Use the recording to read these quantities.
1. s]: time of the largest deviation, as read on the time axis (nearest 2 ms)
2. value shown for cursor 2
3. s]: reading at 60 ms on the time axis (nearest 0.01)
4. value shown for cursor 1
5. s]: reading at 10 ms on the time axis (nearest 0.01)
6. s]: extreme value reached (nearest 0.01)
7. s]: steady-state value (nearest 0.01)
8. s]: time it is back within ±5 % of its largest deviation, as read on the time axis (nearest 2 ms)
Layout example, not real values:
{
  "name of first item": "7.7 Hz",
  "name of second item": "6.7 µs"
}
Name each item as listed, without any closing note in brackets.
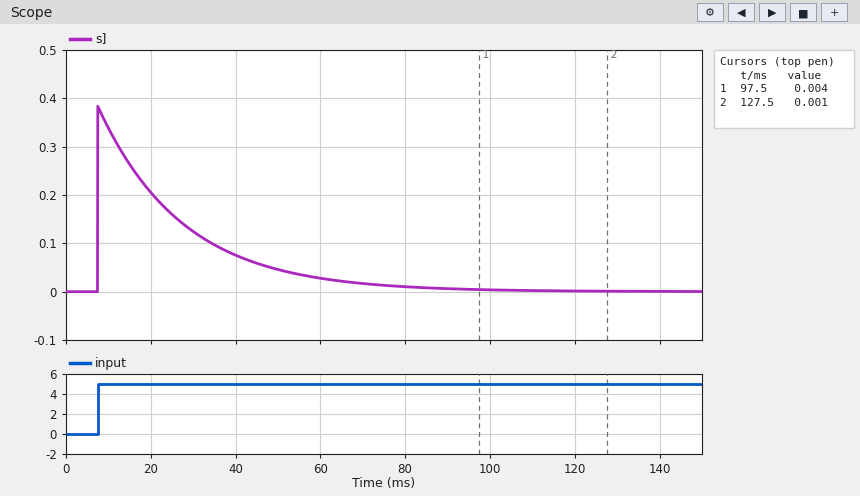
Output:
{
  "s]: time of the largest deviation, as read on the time axis": "8 ms",
  "value shown for cursor 2": "0.001",
  "s]: reading at 60 ms on the time axis": "0.03",
  "value shown for cursor 1": "0.004",
  "s]: reading at 10 ms on the time axis": "0.34",
  "s]: extreme value reached": "0.38",
  "s]: steady-state value": "0.00",
  "s]: time it is back within ±5 % of its largest deviation, as read on the time axis": "68 ms"
}
